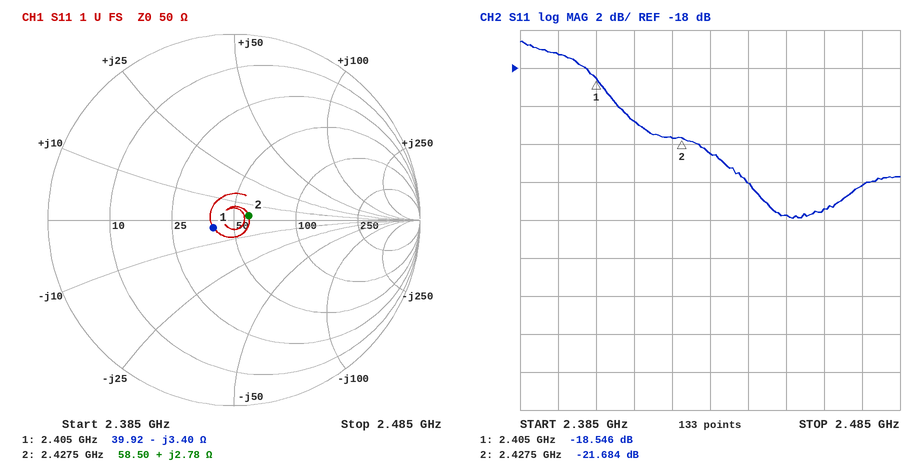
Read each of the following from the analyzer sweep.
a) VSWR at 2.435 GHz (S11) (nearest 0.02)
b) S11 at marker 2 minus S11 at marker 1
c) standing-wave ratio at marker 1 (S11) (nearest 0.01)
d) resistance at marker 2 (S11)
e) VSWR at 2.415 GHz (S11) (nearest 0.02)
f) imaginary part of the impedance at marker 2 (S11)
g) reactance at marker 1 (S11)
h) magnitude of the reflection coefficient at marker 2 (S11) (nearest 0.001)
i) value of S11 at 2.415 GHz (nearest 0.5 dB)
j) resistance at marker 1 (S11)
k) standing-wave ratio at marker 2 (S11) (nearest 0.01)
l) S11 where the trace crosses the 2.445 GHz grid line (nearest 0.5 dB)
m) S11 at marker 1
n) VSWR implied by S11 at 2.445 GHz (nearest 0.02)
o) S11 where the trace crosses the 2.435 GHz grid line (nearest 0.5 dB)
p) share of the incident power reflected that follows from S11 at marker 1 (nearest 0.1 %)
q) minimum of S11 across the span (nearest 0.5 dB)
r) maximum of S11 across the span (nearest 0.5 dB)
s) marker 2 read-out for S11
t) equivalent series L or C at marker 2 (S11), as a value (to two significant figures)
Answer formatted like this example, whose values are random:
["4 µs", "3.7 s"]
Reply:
["1.16", "-3.138 dB", "1.27", "58.50 Ω", "1.20", "+2.78 Ω", "-3.40 Ω", "0.082", "-21.0 dB", "39.92 Ω", "1.18", "-24.0 dB", "-18.546 dB", "1.14", "-22.5 dB", "1.4 %", "-26.0 dB", "-16.5 dB", "-21.684 dB", "180 pH"]
